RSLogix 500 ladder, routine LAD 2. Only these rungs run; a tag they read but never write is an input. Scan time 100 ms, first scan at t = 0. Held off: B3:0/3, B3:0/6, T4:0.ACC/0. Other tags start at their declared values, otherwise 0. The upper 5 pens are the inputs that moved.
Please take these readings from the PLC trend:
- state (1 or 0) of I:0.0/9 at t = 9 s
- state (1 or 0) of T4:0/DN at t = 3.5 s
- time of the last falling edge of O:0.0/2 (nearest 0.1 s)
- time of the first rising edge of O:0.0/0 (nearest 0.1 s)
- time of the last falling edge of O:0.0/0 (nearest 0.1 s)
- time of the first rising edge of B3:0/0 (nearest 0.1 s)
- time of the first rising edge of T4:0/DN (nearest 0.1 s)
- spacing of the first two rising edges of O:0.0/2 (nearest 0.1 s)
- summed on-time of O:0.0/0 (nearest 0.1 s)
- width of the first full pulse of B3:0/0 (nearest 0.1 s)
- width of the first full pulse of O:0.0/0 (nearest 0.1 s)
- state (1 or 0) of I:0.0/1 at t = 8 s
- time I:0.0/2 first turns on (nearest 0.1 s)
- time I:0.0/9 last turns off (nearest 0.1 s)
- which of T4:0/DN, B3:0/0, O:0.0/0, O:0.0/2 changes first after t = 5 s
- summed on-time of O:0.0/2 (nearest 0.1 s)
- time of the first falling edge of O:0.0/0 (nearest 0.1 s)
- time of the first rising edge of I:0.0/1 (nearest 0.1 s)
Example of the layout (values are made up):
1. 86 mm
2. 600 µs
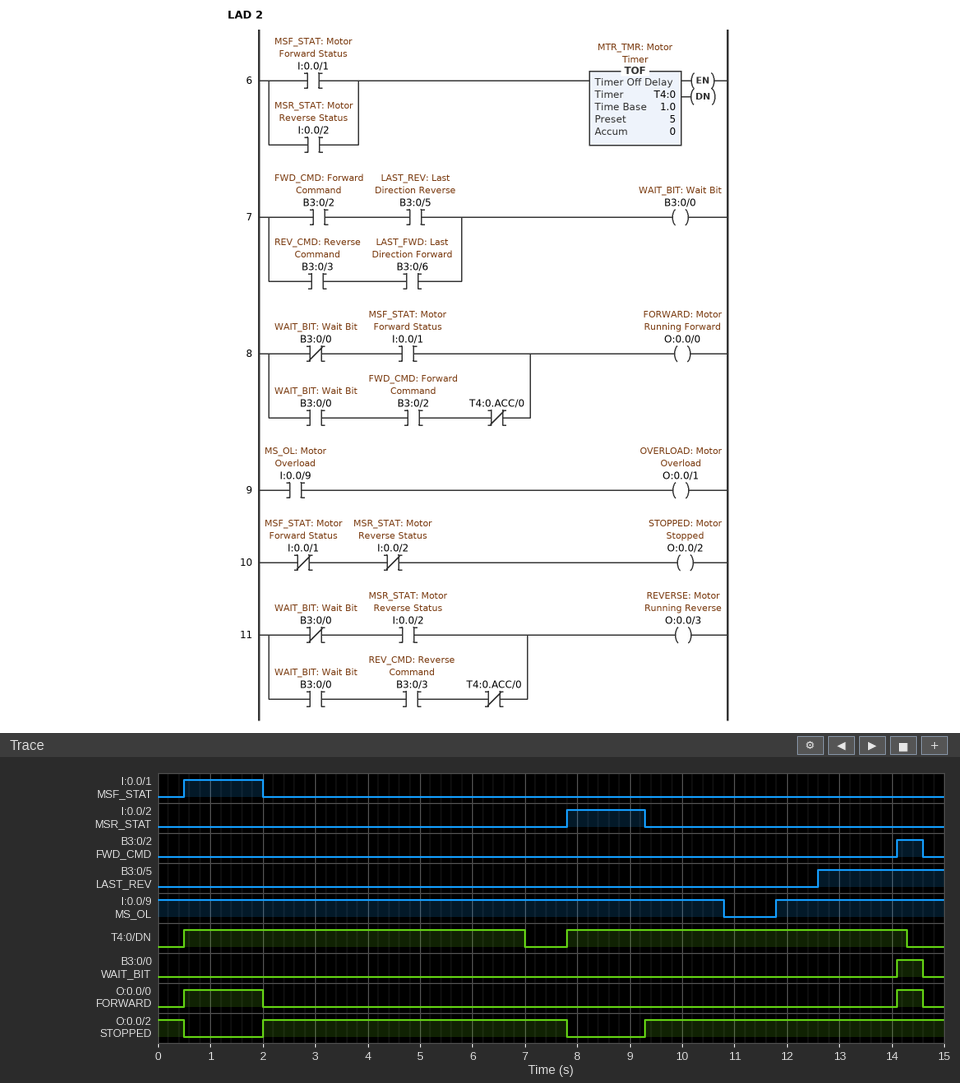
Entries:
1. 1
2. 1
3. 7.8 s
4. 0.5 s
5. 14.6 s
6. 14.1 s
7. 0.5 s
8. 7.3 s
9. 2.0 s
10. 0.5 s
11. 1.5 s
12. 0
13. 7.8 s
14. 10.8 s
15. T4:0/DN
16. 12.0 s
17. 2.0 s
18. 0.5 s
